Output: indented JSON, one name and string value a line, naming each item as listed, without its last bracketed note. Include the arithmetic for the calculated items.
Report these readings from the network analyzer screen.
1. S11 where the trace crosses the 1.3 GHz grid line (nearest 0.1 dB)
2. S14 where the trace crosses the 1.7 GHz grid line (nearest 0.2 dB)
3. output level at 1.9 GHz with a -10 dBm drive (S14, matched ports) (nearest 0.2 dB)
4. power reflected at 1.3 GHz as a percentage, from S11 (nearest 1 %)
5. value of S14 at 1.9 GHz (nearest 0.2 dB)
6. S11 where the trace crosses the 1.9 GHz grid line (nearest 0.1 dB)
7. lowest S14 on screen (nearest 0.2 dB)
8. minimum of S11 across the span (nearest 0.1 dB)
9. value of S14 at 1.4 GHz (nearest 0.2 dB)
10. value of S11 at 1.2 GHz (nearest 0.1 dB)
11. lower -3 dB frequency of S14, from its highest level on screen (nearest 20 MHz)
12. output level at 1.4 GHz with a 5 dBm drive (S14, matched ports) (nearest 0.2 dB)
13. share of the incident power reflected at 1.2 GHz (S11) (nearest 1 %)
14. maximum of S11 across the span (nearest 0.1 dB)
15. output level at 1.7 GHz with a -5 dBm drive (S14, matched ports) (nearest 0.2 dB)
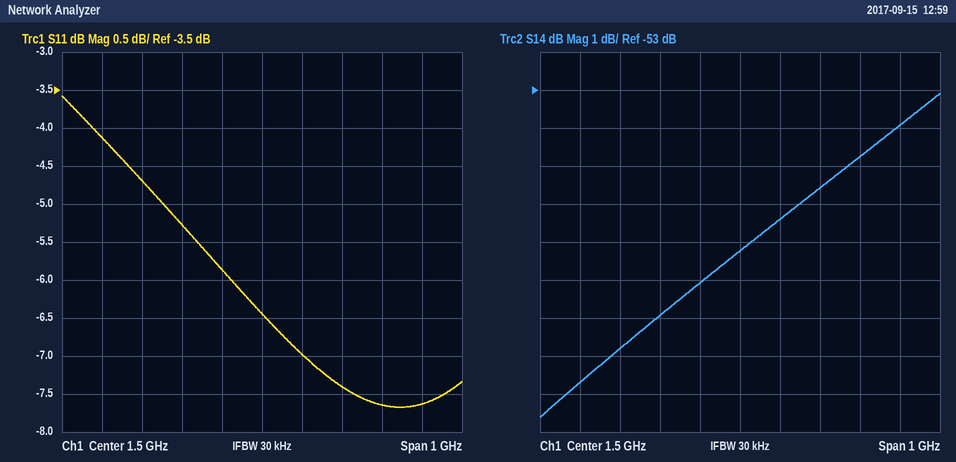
{
  "S11 where the trace crosses the 1.3 GHz grid line": "-5.3 dB",
  "S14 where the trace crosses the 1.7 GHz grid line": "-55.6 dB",
  "output level at 1.9 GHz with a -10 dBm drive (S14, matched ports)": "-10 dBm + (-54.0 dB) = -64.0 dBm",
  "power reflected at 1.3 GHz as a percentage, from S11": "10^(-5.3/10) ≈ 30 %",
  "value of S14 at 1.9 GHz": "-54.0 dB",
  "S11 where the trace crosses the 1.9 GHz grid line": "-7.6 dB",
  "lowest S14 on screen": "-61.6 dB",
  "minimum of S11 across the span": "-7.7 dB",
  "value of S14 at 1.4 GHz": "-58.0 dB",
  "value of S11 at 1.2 GHz": "-4.7 dB",
  "lower -3 dB frequency of S14, from its highest level on screen": "1.64 GHz",
  "output level at 1.4 GHz with a 5 dBm drive (S14, matched ports)": "5 dBm + (-58.0 dB) = -53.0 dBm",
  "share of the incident power reflected at 1.2 GHz (S11)": "10^(-4.7/10) ≈ 34 %",
  "maximum of S11 across the span": "-3.6 dB",
  "output level at 1.7 GHz with a -5 dBm drive (S14, matched ports)": "-5 dBm + (-55.6 dB) = -60.6 dBm"
}
